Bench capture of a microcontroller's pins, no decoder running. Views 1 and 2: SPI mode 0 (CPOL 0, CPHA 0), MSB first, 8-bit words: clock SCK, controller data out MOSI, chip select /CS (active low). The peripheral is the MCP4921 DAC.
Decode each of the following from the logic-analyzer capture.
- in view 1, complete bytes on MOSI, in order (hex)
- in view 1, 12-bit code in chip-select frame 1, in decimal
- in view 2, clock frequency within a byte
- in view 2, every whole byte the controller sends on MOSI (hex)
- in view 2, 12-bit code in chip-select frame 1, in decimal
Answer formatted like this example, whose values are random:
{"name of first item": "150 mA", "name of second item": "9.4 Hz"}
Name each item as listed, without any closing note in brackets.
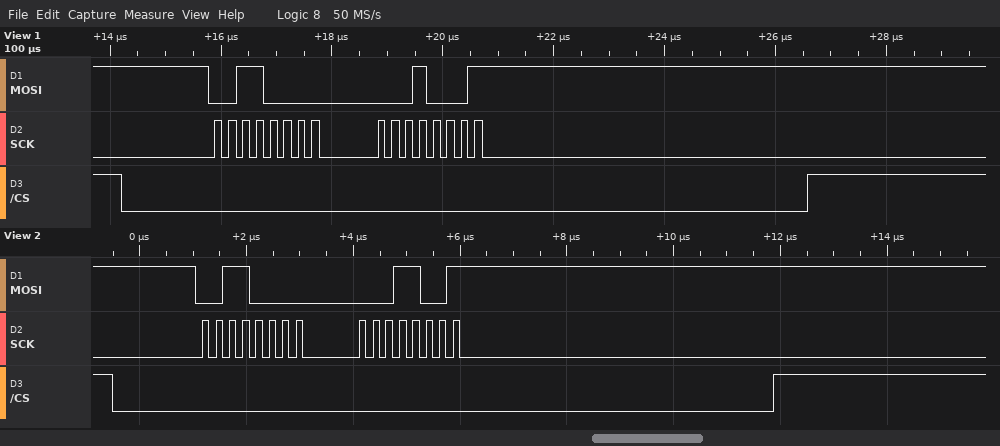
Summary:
{"in view 1, complete bytes on MOSI, in order": "0x30 0x11", "in view 1, 12-bit code in chip-select frame 1, in decimal": "17", "in view 2, clock frequency within a byte": "4 MHz", "in view 2, every whole byte the controller sends on MOSI": "30 19", "in view 2, 12-bit code in chip-select frame 1, in decimal": "25"}
